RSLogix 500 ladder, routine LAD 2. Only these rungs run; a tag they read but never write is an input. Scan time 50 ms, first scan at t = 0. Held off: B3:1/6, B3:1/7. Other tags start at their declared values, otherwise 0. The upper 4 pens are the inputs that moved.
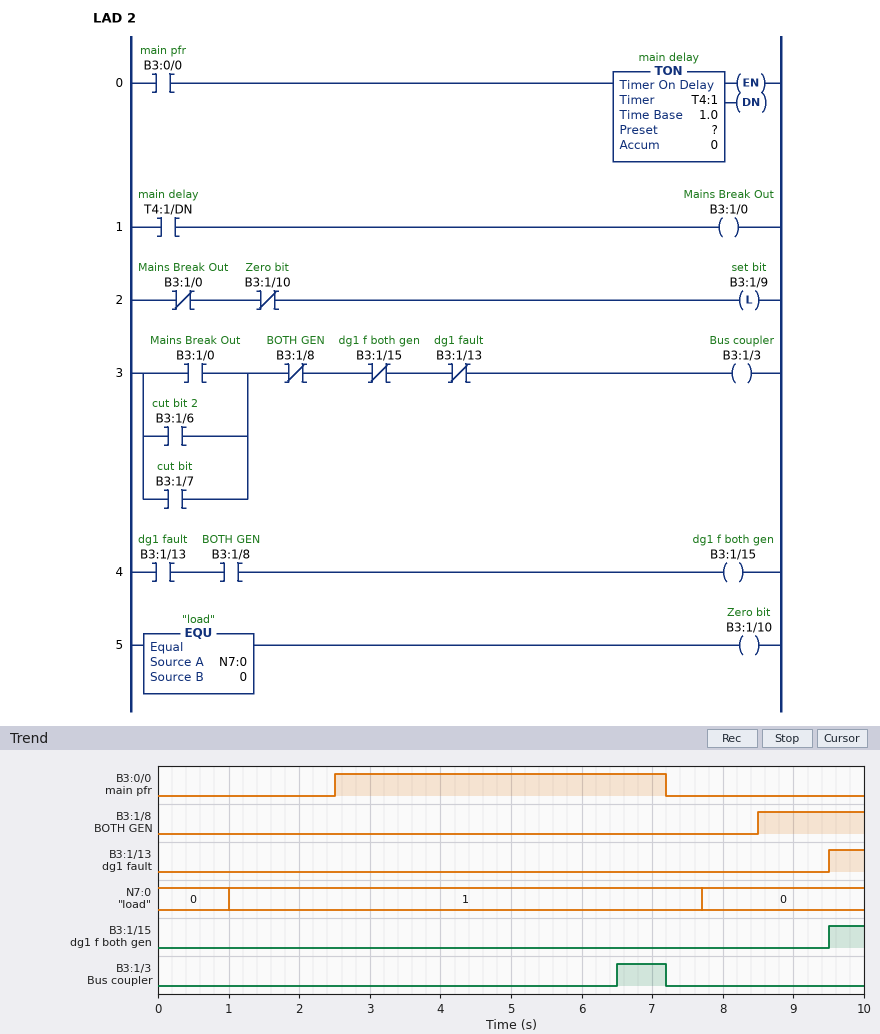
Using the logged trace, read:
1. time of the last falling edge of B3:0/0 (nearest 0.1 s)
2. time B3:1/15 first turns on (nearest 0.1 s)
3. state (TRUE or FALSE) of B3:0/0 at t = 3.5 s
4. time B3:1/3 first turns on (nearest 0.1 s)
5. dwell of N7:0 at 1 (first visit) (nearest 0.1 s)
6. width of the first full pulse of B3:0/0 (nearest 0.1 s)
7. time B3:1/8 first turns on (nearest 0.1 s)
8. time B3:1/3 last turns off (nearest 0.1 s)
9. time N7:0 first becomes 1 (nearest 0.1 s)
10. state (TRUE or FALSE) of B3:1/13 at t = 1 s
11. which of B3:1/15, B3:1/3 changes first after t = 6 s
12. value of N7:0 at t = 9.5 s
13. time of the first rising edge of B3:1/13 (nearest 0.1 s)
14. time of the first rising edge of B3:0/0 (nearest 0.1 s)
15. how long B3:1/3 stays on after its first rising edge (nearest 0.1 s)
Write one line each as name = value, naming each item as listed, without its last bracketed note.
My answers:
time of the last falling edge of B3:0/0 = 7.2 s
time B3:1/15 first turns on = 9.5 s
state (TRUE or FALSE) of B3:0/0 at t = 3.5 s = TRUE
time B3:1/3 first turns on = 6.5 s
dwell of N7:0 at 1 (first visit) = 6.7 s
width of the first full pulse of B3:0/0 = 4.7 s
time B3:1/8 first turns on = 8.5 s
time B3:1/3 last turns off = 7.2 s
time N7:0 first becomes 1 = 1.0 s
state (TRUE or FALSE) of B3:1/13 at t = 1 s = FALSE
which of B3:1/15, B3:1/3 changes first after t = 6 s = B3:1/3
value of N7:0 at t = 9.5 s = 0
time of the first rising edge of B3:1/13 = 9.5 s
time of the first rising edge of B3:0/0 = 2.5 s
how long B3:1/3 stays on after its first rising edge = 0.7 s
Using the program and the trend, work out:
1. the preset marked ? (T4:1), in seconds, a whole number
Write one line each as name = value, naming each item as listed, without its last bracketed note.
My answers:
the preset marked ? (T4:1), in seconds, a whole number = 4 s
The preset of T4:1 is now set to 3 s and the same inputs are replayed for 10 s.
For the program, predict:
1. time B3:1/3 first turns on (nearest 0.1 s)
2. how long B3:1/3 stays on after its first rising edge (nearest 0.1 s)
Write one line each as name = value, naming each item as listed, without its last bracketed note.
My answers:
time B3:1/3 first turns on = 5.5 s
how long B3:1/3 stays on after its first rising edge = 1.7 s
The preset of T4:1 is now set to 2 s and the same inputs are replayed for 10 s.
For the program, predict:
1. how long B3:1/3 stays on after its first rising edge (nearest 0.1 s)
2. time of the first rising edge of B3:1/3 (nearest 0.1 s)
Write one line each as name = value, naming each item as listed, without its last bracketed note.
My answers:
how long B3:1/3 stays on after its first rising edge = 2.7 s
time of the first rising edge of B3:1/3 = 4.5 s
